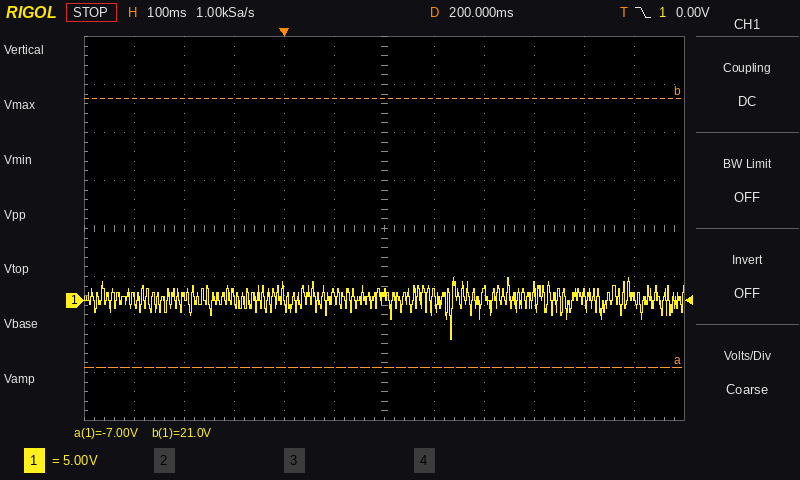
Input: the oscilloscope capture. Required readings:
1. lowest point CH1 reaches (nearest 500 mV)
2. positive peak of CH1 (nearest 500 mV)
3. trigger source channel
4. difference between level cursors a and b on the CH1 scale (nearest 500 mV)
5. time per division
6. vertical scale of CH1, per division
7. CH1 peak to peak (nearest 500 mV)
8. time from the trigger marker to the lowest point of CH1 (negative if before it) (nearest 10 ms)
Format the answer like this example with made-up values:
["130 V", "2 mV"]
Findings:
["-4.0 V", "2.5 V", "CH1", "28.0 V", "100 ms", "5 V", "6.5 V", "+330 ms"]
